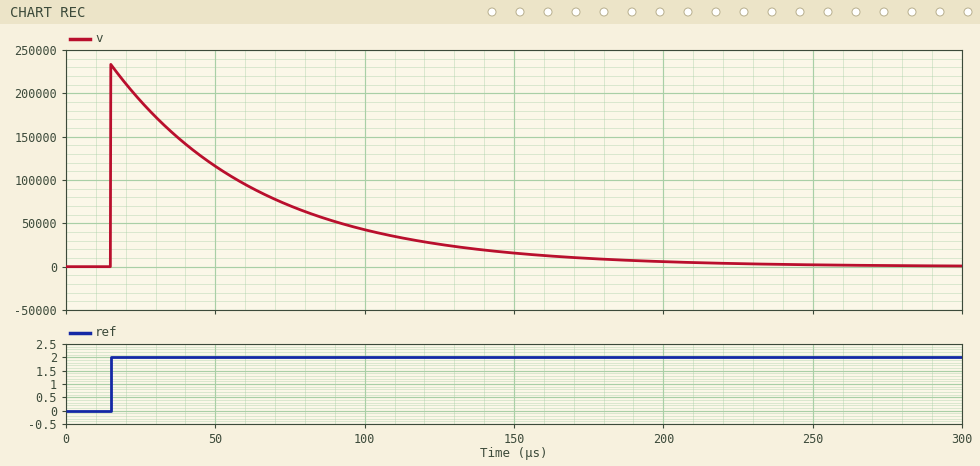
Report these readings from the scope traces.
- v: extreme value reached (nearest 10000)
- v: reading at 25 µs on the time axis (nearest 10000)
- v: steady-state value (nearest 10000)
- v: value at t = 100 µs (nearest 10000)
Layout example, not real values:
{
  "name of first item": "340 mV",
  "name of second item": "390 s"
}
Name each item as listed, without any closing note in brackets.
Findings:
{
  "v: extreme value reached": "230000",
  "v: reading at 25 µs on the time axis": "190000",
  "v: steady-state value": "0",
  "v: value at t = 100 µs": "40000"
}
